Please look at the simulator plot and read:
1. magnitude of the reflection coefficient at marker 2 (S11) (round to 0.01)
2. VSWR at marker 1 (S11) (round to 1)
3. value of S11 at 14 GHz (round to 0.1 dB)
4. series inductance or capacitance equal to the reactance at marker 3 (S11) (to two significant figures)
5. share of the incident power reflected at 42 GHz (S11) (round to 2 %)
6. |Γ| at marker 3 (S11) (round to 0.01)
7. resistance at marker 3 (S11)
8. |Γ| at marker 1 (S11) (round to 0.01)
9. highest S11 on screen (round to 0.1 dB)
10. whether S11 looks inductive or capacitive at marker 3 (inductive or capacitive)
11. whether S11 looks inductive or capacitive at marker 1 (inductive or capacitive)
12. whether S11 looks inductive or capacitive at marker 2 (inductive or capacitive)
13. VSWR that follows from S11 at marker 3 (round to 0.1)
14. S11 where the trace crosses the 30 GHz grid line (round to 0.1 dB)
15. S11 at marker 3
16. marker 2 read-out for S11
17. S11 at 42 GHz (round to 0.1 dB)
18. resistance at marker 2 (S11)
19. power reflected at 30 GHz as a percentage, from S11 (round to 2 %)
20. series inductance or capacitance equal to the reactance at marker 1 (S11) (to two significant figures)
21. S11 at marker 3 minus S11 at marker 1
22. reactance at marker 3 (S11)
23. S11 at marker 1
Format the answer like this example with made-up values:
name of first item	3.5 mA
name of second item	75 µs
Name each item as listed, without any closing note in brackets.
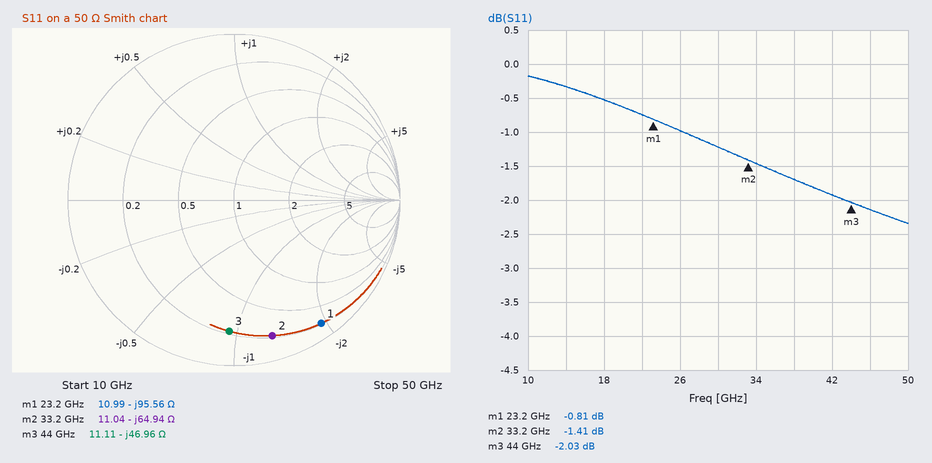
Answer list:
magnitude of the reflection coefficient at marker 2 (S11)	0.85
VSWR at marker 1 (S11)	21
value of S11 at 14 GHz	-0.3 dB
series inductance or capacitance equal to the reactance at marker 3 (S11)	77 fF
share of the incident power reflected at 42 GHz (S11)	64 %
|Γ| at marker 3 (S11)	0.79
resistance at marker 3	11.11 Ω
|Γ| at marker 1 (S11)	0.91
highest S11 on screen	-0.2 dB
whether S11 looks inductive or capacitive at marker 3	capacitive
whether S11 looks inductive or capacitive at marker 1	capacitive
whether S11 looks inductive or capacitive at marker 2	capacitive
VSWR that follows from S11 at marker 3	8.6
S11 where the trace crosses the 30 GHz grid line	-1.2 dB
S11 at marker 3	-2.03 dB
marker 2 read-out for S11	-1.41 dB
S11 at 42 GHz	-1.9 dB
resistance at marker 2	11.04 Ω
power reflected at 30 GHz as a percentage, from S11	76 %
series inductance or capacitance equal to the reactance at marker 1 (S11)	72 fF
S11 at marker 3 minus S11 at marker 1	-1.22 dB
reactance at marker 3	-46.96 Ω
S11 at marker 1	-0.81 dB
